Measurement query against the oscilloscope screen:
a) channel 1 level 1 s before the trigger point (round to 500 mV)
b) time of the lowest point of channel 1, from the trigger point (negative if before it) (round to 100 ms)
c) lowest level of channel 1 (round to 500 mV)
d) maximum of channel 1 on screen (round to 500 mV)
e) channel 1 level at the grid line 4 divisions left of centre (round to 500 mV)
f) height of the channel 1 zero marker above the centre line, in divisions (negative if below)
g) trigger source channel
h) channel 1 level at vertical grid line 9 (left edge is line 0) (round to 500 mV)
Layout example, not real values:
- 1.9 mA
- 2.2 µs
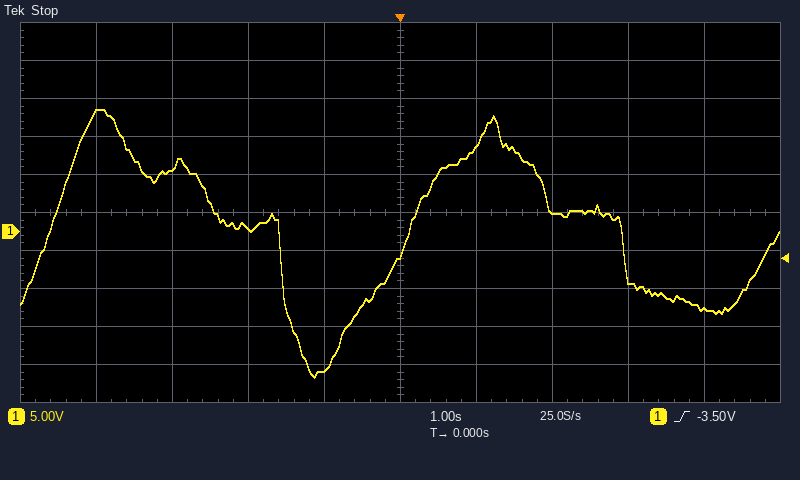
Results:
- -18.0 V
- -1.1 s
- -19.0 V
- 16.0 V
- 15.5 V
- -0.5 div
- channel 1
- -10.0 V
